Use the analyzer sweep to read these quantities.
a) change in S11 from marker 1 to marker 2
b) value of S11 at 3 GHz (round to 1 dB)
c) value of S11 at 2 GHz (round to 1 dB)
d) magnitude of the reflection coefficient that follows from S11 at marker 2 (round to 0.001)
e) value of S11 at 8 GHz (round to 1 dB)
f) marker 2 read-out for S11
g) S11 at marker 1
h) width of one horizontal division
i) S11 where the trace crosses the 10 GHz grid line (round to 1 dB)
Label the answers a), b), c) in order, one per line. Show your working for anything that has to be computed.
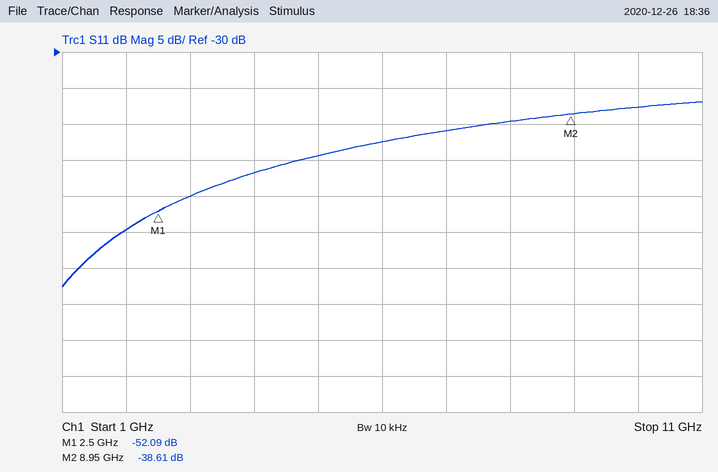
a) -38.61 − (-52.09) = 13.48 dB
b) -50 dB
c) -55 dB
d) 10^(-38.61/20) ≈ 0.012
e) -40 dB
f) -38.61 dB
g) -52.09 dB
h) 1 GHz
i) -38 dB
